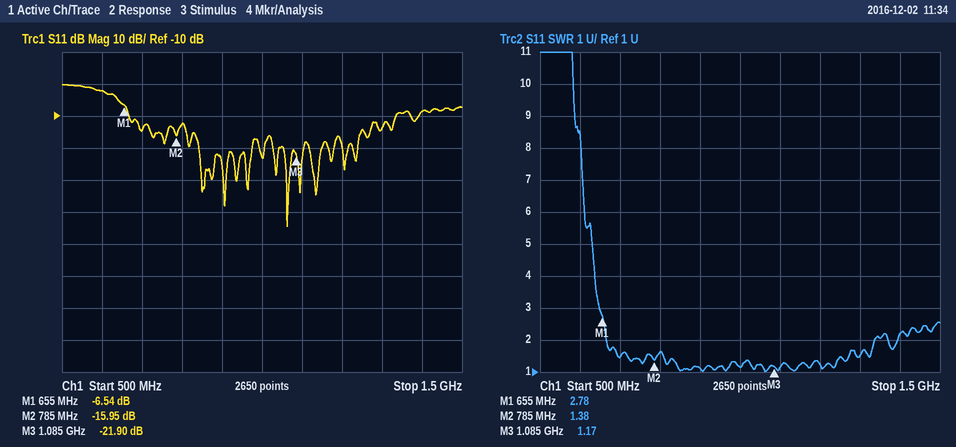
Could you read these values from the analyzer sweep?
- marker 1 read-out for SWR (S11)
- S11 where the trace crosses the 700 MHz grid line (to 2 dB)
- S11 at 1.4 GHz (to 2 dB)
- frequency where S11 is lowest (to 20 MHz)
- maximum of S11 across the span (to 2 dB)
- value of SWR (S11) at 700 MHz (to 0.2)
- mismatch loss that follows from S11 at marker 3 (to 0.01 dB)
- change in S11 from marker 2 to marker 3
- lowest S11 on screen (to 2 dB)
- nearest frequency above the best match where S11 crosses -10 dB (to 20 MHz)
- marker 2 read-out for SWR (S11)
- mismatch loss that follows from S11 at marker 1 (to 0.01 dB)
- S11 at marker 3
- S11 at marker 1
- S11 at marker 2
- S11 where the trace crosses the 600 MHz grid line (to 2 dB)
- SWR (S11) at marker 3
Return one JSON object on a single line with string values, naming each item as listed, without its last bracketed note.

{"marker 1 read-out for SWR": "2.78", "S11 where the trace crosses the 700 MHz grid line": "-14 dB", "S11 at 1.4 GHz": "-8 dB", "frequency where S11 is lowest": "1.06 GHz", "maximum of S11 across the span": "0 dB", "value of SWR (S11) at 700 MHz": "1.4", "mismatch loss that follows from S11 at marker 3": "0.03 dB", "change in S11 from marker 2 to marker 3": "-5.95 dB", "lowest S11 on screen": "-44 dB", "nearest frequency above the best match where S11 crosses -10 dB": "1.34 GHz", "marker 2 read-out for SWR": "1.38", "mismatch loss that follows from S11 at marker 1": "1.09 dB", "S11 at marker 3": "-21.90 dB", "S11 at marker 1": "-6.54 dB", "S11 at marker 2": "-15.95 dB", "S11 where the trace crosses the 600 MHz grid line": "-2 dB", "SWR (S11) at marker 3": "1.17"}
